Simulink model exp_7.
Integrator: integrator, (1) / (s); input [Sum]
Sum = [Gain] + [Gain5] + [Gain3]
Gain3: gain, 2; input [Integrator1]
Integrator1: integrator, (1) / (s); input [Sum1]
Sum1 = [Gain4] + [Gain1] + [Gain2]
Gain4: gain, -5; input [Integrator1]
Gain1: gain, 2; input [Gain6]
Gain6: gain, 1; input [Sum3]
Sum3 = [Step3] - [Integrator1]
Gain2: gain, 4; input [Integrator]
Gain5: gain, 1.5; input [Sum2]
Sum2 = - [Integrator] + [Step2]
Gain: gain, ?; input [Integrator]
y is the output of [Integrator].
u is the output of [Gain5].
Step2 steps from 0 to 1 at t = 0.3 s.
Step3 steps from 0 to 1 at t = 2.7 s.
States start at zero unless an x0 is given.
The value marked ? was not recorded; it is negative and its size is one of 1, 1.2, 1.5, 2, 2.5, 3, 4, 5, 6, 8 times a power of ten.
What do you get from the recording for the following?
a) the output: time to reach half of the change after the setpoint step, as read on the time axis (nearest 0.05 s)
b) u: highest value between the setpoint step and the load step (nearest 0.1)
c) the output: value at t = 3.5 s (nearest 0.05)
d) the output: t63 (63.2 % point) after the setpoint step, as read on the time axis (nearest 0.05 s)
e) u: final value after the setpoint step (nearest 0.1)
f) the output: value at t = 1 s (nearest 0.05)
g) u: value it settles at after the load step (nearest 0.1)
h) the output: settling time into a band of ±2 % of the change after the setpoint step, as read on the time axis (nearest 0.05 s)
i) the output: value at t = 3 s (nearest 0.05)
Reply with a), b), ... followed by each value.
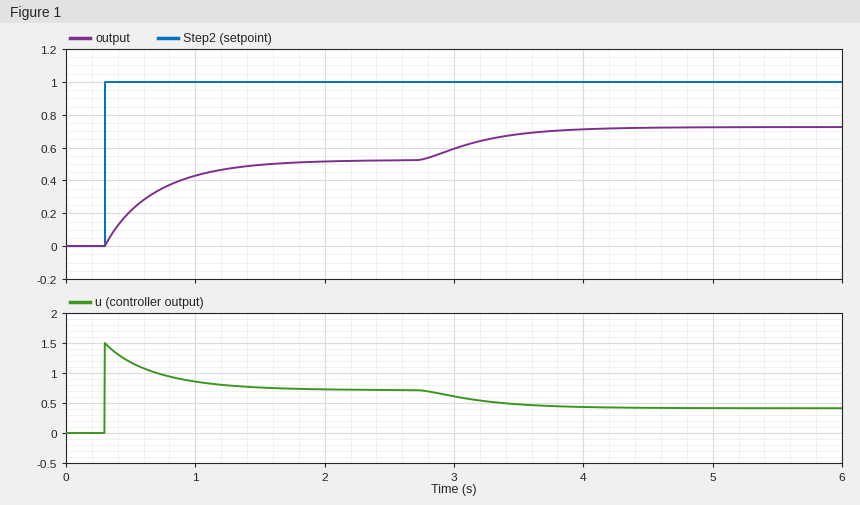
a) 0.55 s
b) 1.5
c) 0.70
d) 0.70 s
e) 0.7
f) 0.45
g) 0.4
h) 1.95 s
i) 0.60
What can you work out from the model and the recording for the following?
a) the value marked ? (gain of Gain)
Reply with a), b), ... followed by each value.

a) -2.5
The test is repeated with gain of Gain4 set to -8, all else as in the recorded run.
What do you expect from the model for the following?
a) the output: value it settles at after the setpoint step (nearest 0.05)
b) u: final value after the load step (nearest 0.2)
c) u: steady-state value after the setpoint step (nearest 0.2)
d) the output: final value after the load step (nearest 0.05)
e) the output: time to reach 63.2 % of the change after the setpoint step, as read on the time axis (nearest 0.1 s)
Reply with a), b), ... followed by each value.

a) 0.45
b) 0.6
c) 0.8
d) 0.60
e) 0.6 s
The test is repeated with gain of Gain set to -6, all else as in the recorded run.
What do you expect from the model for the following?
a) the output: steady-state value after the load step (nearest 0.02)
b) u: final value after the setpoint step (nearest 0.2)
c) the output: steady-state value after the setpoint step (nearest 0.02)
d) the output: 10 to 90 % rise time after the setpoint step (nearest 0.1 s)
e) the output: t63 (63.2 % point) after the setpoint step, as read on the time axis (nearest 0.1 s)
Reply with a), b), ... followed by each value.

a) 0.32
b) 1.2
c) 0.24
d) 0.4 s
e) 0.5 s
